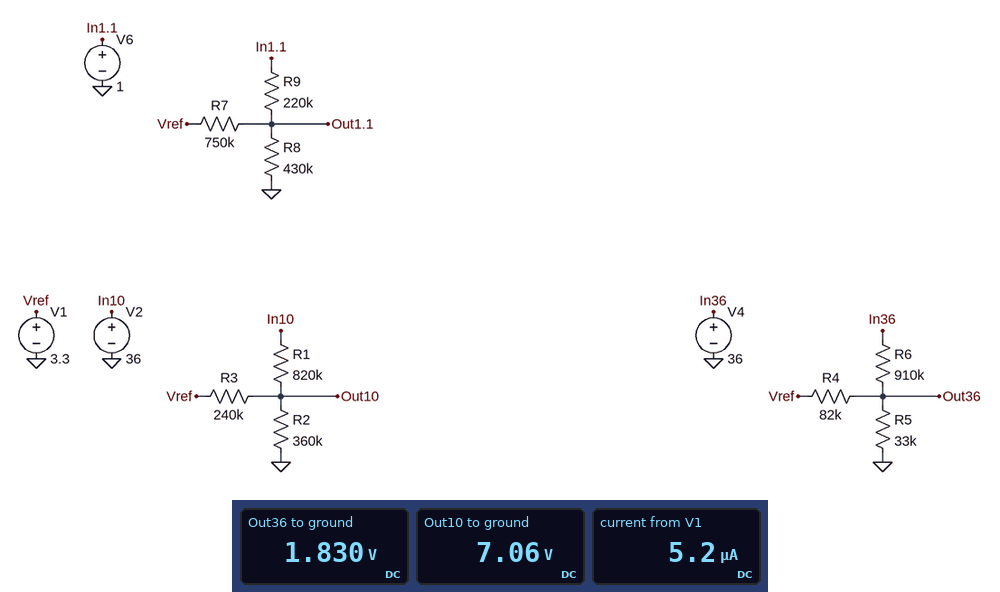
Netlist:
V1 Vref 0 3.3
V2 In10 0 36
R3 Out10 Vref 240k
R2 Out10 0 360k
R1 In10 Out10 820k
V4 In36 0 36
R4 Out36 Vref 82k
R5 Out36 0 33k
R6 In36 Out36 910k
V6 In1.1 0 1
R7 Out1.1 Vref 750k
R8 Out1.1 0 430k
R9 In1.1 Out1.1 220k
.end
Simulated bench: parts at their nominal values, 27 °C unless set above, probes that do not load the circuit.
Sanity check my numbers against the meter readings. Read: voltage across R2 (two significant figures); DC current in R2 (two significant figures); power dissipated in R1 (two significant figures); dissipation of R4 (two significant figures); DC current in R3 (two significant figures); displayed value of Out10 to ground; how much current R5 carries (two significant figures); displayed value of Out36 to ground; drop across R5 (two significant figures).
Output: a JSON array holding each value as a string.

["7.1 V", "20 µA", "1.0 mW", "26 µW", "16 µA", "7.06 V", "55 µA", "1.830 V", "1.8 V"]
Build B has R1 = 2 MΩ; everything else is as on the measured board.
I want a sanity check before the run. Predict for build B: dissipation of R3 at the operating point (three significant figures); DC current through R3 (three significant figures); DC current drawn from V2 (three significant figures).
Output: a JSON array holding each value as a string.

["3.88 µW", "4.02 µA", "15.9 µA"]
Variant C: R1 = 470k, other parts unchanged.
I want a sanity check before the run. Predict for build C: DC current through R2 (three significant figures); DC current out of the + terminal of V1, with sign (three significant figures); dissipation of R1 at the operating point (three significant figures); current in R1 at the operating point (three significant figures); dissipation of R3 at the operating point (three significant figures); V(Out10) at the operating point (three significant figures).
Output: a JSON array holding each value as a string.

["27.7 µA", "-6.88 µA", "1.44 mW", "55.4 µA", "185 µW", "9.96 V"]
